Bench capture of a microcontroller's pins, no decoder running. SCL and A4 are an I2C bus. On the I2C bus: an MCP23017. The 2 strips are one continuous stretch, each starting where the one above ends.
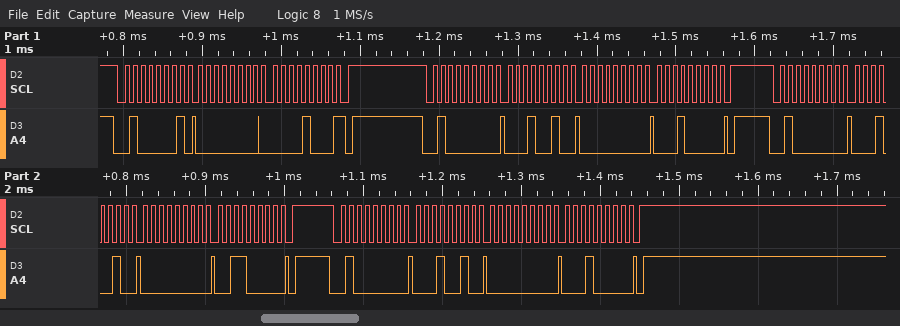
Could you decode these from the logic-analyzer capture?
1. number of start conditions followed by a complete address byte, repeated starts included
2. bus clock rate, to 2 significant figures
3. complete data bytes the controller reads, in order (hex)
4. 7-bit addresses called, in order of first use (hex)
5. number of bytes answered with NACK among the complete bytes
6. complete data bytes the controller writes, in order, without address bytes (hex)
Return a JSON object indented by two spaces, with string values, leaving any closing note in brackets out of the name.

{
  "number of start conditions followed by a complete address byte, repeated starts included": "4",
  "bus clock rate, to 2 significant figures": "100 kHz",
  "complete data bytes the controller reads, in order": "00 08",
  "7-bit addresses called, in order of first use": "0x20",
  "number of bytes answered with NACK among the complete bytes": "1",
  "complete data bytes the controller writes, in order, without address bytes": "12 00 10 12 00 30 12 00 10"
}
